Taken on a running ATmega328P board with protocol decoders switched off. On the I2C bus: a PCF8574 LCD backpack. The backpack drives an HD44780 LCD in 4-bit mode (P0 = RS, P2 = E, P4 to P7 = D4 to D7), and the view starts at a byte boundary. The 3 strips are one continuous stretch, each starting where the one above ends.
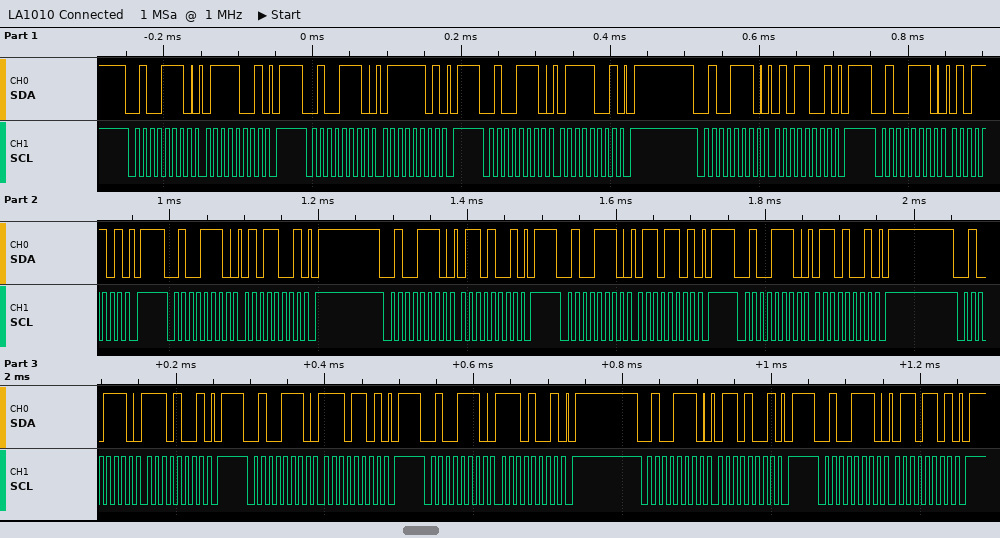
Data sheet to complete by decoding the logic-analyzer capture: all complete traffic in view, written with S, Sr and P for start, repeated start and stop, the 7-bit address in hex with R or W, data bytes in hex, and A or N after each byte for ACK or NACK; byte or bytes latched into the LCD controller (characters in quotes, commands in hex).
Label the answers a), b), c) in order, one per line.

a) S 27W A 79 A P S 27W A 7D A P S 27W A 79 A P S 27W A 59 A P S 27W A 5D A P S 27W A 59 A P S 27W A 69 A P S 27W A 6D A P S 27W A 69 A P S 27W A E9 A P S 27W A ED A P S 27W A E9 A P S 27W A 69 A P S 27W A 6D A P
b) 'u' 'n'
